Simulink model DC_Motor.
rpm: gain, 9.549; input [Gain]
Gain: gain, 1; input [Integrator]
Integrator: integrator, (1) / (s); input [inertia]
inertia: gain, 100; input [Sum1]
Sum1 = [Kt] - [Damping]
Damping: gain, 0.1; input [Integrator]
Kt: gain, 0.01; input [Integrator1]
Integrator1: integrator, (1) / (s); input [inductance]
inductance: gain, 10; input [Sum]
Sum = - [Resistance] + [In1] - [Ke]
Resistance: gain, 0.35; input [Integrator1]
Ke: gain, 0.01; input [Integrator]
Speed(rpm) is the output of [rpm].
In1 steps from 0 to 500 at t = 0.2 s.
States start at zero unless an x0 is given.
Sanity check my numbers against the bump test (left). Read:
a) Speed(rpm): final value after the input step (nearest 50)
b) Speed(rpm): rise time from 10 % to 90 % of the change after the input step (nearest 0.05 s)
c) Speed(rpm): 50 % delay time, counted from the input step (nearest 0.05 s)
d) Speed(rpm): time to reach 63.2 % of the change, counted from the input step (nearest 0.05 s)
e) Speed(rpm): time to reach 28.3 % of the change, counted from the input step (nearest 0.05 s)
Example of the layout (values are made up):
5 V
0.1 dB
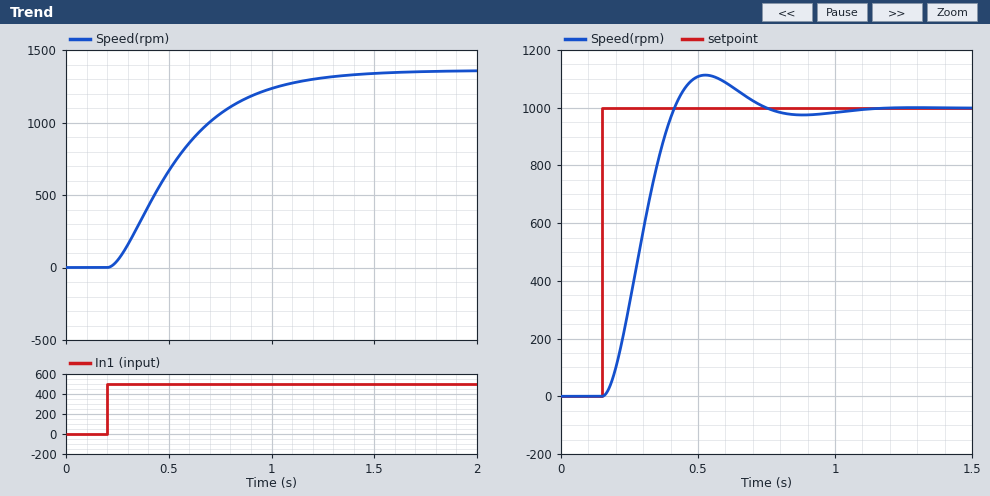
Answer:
1350
0.70 s
0.30 s
0.40 s
0.20 s
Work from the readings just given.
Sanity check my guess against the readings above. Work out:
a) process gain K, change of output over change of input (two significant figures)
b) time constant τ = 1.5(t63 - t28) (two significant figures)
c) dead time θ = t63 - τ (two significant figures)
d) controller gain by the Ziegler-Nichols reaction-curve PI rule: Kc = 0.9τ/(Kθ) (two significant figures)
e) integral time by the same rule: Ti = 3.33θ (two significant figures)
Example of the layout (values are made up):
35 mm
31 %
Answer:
2.7
0.30 s
0.10 s
1.0
0.33 s
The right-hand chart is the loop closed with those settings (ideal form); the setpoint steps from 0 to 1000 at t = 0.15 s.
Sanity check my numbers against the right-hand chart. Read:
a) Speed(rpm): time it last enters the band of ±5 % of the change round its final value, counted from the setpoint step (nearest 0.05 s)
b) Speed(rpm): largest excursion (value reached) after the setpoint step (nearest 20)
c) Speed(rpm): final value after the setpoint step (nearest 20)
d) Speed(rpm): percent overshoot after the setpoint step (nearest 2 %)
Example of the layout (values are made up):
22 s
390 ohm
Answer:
0.50 s
1120
1000
12 %
